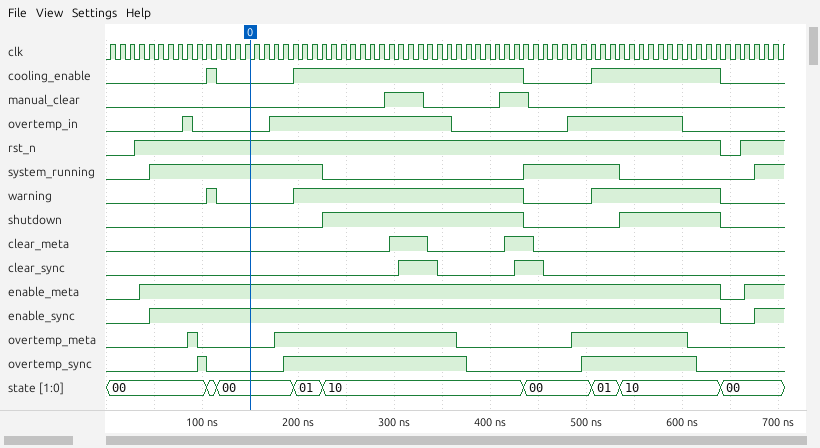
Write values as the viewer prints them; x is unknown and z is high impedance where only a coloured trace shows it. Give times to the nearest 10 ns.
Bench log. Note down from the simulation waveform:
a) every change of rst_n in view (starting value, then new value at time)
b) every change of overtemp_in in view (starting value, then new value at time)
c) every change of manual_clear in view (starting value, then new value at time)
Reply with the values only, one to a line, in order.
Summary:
0, 1 at 30 ns, 0 at 640 ns, 1 at 660 ns
0, 1 at 80 ns, 0 at 90 ns, 1 at 170 ns, 0 at 360 ns, 1 at 480 ns, 0 at 600 ns
0, 1 at 290 ns, 0 at 330 ns, 1 at 410 ns, 0 at 440 ns
